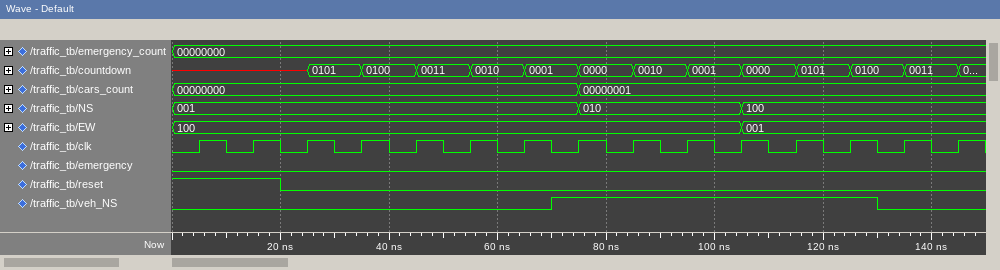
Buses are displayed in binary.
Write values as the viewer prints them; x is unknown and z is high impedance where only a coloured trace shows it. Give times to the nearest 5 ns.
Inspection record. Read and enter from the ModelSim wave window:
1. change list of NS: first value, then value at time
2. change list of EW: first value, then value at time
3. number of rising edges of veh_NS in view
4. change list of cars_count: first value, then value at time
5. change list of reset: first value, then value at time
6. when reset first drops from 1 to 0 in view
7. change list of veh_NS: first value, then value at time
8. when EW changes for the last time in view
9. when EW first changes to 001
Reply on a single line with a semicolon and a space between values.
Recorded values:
001, 010 at 75 ns, 100 at 105 ns; 100, 001 at 105 ns; 1; 00000000, 00000001 at 75 ns; 1, 0 at 20 ns; 20 ns; 0, 1 at 70 ns, 0 at 130 ns; 105 ns; 105 ns
